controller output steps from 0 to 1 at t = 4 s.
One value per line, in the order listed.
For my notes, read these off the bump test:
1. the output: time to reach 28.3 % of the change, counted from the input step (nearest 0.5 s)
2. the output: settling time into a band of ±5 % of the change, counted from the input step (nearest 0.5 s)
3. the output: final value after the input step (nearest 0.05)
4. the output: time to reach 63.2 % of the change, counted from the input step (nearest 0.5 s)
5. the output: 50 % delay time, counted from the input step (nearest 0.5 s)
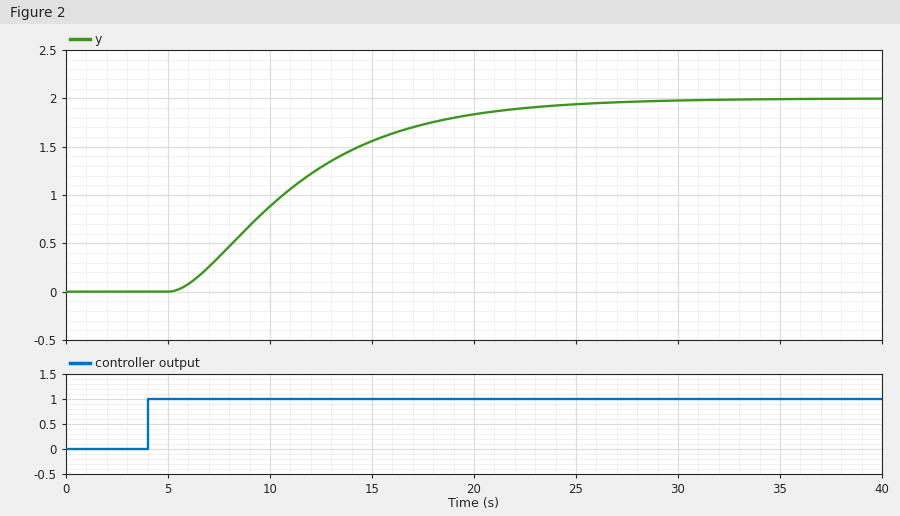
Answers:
4.5 s
18.5 s
2.00
8.5 s
6.5 s
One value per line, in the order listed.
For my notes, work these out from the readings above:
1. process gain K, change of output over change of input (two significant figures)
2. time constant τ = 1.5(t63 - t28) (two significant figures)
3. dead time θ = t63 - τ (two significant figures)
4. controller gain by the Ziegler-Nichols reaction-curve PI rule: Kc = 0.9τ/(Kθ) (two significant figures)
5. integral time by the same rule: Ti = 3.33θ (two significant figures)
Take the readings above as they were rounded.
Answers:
2.0
6.0 s
2.5 s
1.1
8.3 s
